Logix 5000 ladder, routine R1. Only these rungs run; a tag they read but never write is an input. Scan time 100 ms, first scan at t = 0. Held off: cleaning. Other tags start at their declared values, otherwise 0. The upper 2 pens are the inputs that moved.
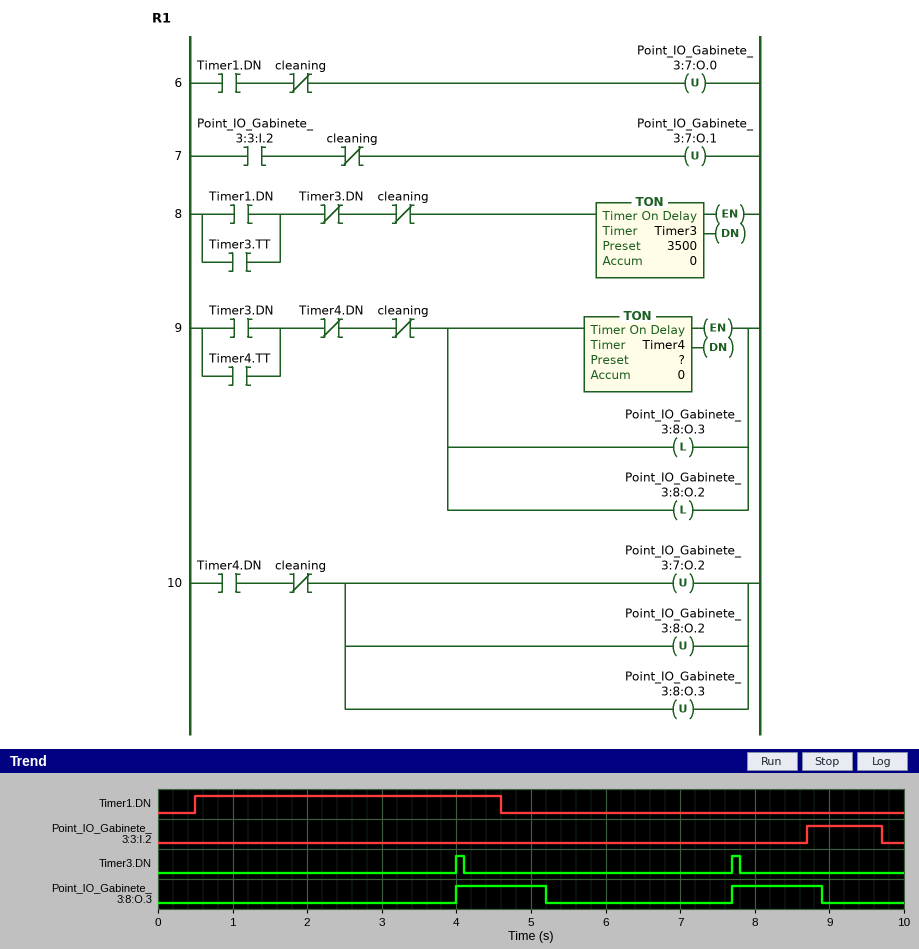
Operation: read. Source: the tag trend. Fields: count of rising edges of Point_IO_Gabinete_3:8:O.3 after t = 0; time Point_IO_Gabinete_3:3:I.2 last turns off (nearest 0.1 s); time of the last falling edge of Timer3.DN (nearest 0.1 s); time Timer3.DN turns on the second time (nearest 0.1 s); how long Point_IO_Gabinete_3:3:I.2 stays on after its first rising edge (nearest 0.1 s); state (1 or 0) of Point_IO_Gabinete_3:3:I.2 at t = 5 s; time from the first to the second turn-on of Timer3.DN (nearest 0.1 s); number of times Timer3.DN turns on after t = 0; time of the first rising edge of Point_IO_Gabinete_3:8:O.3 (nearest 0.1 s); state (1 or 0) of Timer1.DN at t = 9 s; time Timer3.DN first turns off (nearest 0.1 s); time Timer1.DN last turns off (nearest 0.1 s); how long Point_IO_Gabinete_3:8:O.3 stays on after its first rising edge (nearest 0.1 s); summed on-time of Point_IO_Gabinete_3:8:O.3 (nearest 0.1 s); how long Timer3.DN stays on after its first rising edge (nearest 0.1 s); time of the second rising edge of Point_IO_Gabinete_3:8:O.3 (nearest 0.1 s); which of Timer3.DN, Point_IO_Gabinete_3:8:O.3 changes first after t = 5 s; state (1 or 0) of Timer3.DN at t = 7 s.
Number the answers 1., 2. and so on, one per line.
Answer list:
1. 2
2. 9.7 s
3. 7.8 s
4. 7.7 s
5. 1.0 s
6. 0
7. 3.7 s
8. 2
9. 4.0 s
10. 0
11. 4.1 s
12. 4.6 s
13. 1.2 s
14. 2.4 s
15. 0.1 s
16. 7.7 s
17. Point_IO_Gabinete_3:8:O.3
18. 0
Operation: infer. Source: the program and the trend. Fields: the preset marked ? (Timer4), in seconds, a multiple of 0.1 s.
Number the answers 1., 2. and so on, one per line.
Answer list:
1. 1.2 s
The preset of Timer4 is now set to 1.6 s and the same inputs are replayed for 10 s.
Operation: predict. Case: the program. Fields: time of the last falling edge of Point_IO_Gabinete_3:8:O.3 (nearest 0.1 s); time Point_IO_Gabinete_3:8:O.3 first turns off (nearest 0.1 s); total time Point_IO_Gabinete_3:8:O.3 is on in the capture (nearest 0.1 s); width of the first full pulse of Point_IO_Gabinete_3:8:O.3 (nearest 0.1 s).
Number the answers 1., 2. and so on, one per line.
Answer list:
1. 9.3 s
2. 5.6 s
3. 3.2 s
4. 1.6 s
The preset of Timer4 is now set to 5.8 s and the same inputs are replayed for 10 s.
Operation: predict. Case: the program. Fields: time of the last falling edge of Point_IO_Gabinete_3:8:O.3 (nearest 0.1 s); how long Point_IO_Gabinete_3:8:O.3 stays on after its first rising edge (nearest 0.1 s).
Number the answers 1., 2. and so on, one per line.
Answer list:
1. 9.8 s
2. 5.8 s
